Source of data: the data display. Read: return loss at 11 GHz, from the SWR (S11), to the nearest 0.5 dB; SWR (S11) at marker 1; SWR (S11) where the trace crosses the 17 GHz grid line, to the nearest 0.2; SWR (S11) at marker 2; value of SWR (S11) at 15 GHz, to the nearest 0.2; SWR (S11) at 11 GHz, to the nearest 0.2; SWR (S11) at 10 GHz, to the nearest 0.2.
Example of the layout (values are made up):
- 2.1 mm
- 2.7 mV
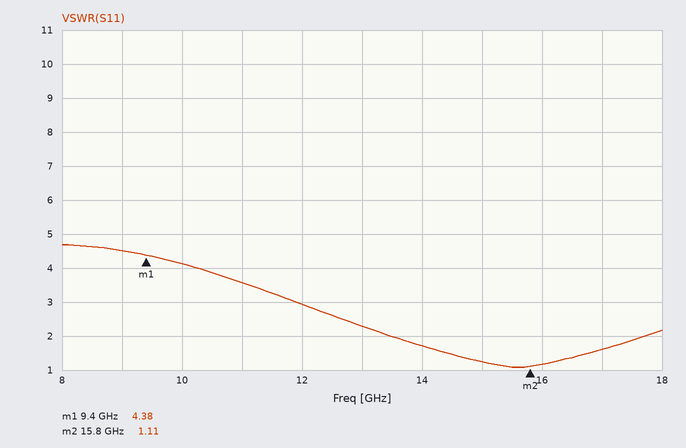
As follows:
- 5.0 dB
- 4.38
- 1.6
- 1.11
- 1.2
- 3.6
- 4.2
